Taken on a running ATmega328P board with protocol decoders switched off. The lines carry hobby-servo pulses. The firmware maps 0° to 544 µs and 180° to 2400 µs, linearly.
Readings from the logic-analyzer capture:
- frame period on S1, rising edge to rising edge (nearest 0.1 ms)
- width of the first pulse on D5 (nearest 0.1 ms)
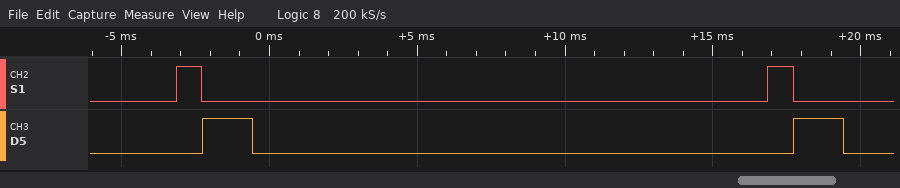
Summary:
20.0 ms
1.7 ms
